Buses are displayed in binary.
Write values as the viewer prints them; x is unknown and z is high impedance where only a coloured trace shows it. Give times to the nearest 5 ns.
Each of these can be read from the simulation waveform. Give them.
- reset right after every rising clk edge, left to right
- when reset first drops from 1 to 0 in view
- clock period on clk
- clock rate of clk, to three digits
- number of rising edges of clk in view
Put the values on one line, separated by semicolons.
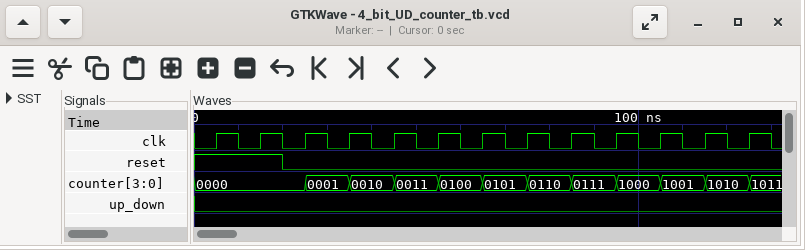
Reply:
1 1 0 0 0 0 0 0 0 0 0 0 0; 20 ns; 10 ns; 100 MHz; 13
